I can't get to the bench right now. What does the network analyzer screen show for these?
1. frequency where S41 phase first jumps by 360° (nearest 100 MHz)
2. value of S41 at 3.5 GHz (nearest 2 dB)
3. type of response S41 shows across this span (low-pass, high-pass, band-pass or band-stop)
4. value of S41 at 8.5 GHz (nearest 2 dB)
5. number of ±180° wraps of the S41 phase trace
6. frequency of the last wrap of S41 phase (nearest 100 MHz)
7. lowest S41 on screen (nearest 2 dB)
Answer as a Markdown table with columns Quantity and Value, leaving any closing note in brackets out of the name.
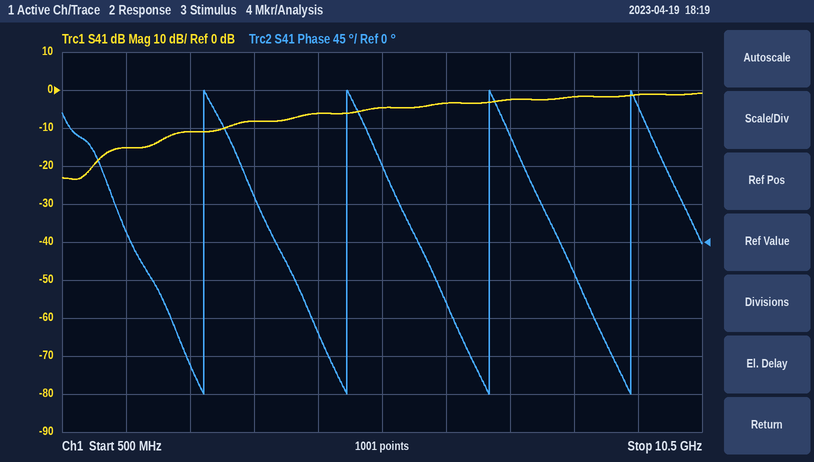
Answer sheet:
| Quantity | Value |
|---|---|
| frequency where S41 phase first jumps by 360° | 2.7 GHz |
| value of S41 at 3.5 GHz | -8 dB |
| type of response S41 shows across this span | high-pass |
| value of S41 at 8.5 GHz | -2 dB |
| number of ±180° wraps of the S41 phase trace | 4 |
| frequency of the last wrap of S41 phase | 9.4 GHz |
| lowest S41 on screen | -24 dB |
